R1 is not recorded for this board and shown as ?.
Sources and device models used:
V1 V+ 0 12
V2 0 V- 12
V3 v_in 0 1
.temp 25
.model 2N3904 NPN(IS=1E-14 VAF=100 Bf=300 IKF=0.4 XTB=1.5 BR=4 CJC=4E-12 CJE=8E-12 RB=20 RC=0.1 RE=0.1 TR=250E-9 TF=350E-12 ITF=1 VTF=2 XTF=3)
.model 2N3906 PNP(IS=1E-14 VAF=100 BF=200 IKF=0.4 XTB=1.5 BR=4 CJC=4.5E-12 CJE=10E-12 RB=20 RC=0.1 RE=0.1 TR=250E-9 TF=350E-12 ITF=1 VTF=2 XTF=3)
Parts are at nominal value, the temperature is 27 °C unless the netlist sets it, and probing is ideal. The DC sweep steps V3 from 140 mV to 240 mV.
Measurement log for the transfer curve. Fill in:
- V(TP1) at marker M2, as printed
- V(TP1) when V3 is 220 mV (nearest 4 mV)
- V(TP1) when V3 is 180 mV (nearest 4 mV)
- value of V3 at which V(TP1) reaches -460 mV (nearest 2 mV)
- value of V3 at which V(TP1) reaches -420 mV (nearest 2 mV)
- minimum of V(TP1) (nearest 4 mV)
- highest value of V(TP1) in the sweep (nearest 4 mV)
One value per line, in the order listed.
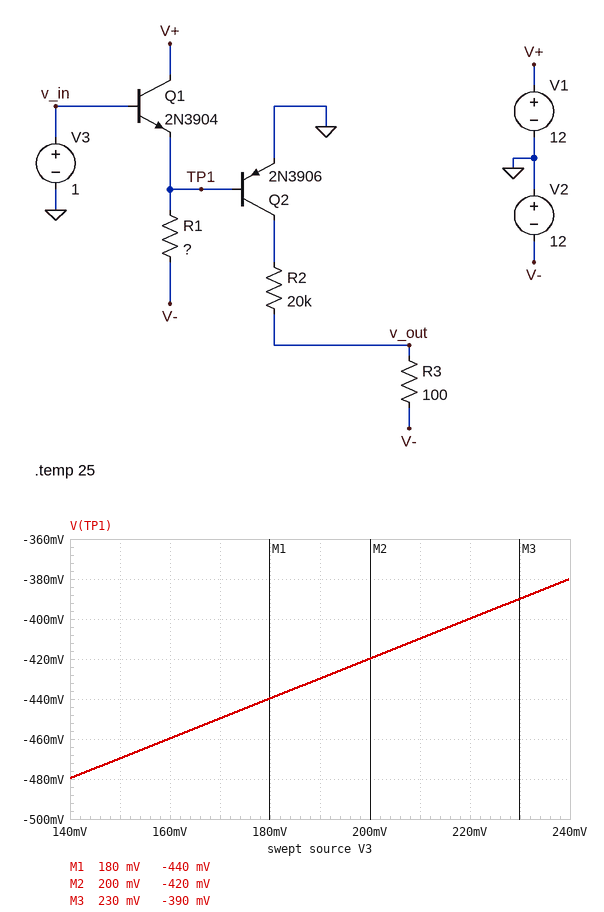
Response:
-420 mV
-400 mV
-440 mV
160 mV
200 mV
-480 mV
-380 mV
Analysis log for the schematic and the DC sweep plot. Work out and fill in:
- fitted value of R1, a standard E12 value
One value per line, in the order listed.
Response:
47 kΩ
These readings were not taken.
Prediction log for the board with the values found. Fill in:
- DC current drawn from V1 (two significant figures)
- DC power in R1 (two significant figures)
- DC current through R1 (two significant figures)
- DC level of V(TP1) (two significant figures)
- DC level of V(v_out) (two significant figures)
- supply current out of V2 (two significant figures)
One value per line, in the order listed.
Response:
260 µA
3.3 mW
260 µA
380 mV
-12 V
260 µA
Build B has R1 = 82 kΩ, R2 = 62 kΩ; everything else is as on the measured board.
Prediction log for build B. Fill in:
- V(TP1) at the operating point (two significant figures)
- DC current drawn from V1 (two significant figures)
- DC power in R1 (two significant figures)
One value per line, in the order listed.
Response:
390 mV
150 µA
1.9 mW
